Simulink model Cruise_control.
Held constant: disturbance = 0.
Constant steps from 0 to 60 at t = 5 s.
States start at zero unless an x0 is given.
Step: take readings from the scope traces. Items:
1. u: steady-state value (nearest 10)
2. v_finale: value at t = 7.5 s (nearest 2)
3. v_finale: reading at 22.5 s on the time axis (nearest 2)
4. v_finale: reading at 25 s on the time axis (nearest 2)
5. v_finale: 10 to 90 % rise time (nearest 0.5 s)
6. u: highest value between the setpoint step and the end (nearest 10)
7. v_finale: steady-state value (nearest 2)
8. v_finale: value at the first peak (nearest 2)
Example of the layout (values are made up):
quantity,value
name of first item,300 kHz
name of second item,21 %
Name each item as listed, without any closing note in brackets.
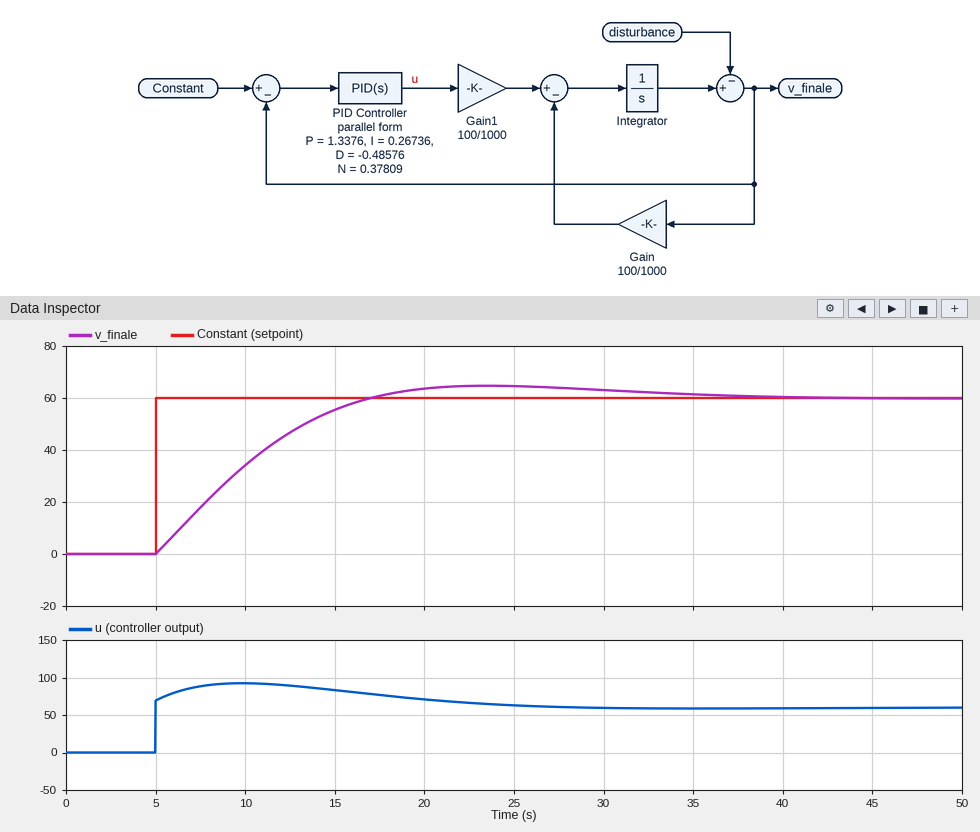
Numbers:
quantity,value
u: steady-state value,60
v_finale: value at t = 7.5 s,18
v_finale: reading at 22.5 s on the time axis,64
v_finale: reading at 25 s on the time axis,64
v_finale: 10 to 90 % rise time,8.5 s
u: highest value between the setpoint step and the end,90
v_finale: steady-state value,60
v_finale: value at the first peak,64
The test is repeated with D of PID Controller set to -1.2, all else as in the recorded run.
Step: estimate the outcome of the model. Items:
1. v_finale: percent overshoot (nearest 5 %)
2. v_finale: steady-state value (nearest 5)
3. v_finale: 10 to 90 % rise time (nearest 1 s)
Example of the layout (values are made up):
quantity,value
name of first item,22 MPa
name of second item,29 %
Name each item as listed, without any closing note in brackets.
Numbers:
quantity,value
v_finale: percent overshoot,10 %
v_finale: steady-state value,60
v_finale: 10 to 90 % rise time,8 s
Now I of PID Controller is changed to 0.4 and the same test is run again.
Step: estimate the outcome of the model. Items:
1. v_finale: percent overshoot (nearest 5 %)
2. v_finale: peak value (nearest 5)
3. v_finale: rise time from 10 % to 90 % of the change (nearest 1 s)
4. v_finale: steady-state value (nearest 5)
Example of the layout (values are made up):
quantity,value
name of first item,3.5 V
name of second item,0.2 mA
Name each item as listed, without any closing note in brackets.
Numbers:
quantity,value
v_finale: percent overshoot,15 %
v_finale: peak value,70
v_finale: rise time from 10 % to 90 % of the change,7 s
v_finale: steady-state value,60
